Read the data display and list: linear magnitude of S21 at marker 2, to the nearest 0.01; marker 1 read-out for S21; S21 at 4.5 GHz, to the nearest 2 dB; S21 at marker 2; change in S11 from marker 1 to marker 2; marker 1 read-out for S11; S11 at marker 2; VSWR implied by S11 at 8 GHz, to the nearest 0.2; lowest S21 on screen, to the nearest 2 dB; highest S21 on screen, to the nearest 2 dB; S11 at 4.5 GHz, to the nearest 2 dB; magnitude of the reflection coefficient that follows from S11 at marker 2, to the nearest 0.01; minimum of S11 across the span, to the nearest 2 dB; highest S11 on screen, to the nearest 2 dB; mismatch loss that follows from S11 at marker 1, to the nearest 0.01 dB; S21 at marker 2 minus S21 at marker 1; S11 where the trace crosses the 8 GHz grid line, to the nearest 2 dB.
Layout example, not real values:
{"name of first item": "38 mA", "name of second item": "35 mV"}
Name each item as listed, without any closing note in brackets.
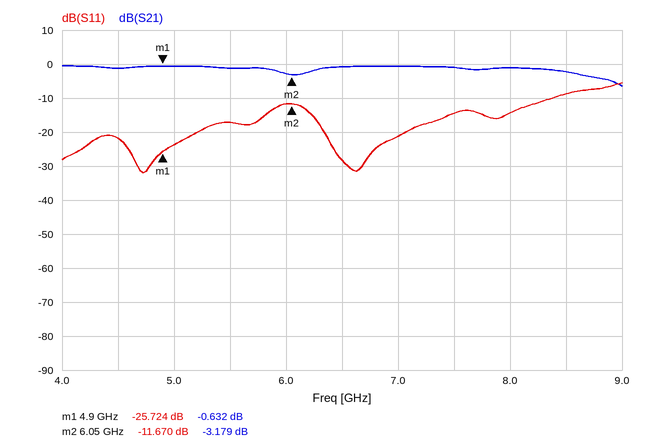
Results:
{"linear magnitude of S21 at marker 2, to the nearest 0.01": "0.69", "marker 1 read-out for S21": "-0.632 dB", "S21 at 4.5 GHz, to the nearest 2 dB": "-2 dB", "S21 at marker 2": "-3.179 dB", "change in S11 from marker 1 to marker 2": "14.054 dB", "marker 1 read-out for S11": "-25.724 dB", "S11 at marker 2": "-11.670 dB", "VSWR implied by S11 at 8 GHz, to the nearest 0.2": "1.4", "lowest S21 on screen, to the nearest 2 dB": "-6 dB", "highest S21 on screen, to the nearest 2 dB": "0 dB", "S11 at 4.5 GHz, to the nearest 2 dB": "-22 dB", "magnitude of the reflection coefficient that follows from S11 at marker 2, to the nearest 0.01": "0.26", "minimum of S11 across the span, to the nearest 2 dB": "-32 dB", "highest S11 on screen, to the nearest 2 dB": "-6 dB", "mismatch loss that follows from S11 at marker 1, to the nearest 0.01 dB": "0.01 dB", "S21 at marker 2 minus S21 at marker 1": "-2.547 dB", "S11 where the trace crosses the 8 GHz grid line, to the nearest 2 dB": "-14 dB"}
